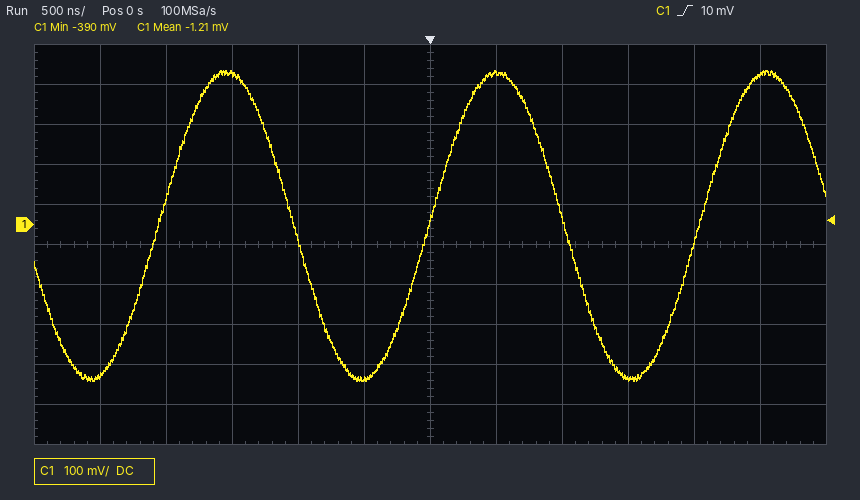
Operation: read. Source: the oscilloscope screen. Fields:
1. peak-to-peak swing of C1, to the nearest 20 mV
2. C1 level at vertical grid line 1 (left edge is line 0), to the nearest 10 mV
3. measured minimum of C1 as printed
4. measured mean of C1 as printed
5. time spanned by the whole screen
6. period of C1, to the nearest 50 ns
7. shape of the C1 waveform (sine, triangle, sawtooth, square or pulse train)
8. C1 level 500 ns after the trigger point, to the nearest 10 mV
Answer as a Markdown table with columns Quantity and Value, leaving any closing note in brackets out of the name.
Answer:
| Quantity | Value |
|---|---|
| peak-to-peak swing of C1, to the nearest 20 mV | 780 mV |
| C1 level at vertical grid line 1 (left edge is line 0), to the nearest 10 mV | -380 mV |
| measured minimum of C1 as printed | -390 mV |
| measured mean of C1 as printed | -1.21 mV |
| time spanned by the whole screen | 6 µs |
| period of C1, to the nearest 50 ns | 2.05 µs |
| shape of the C1 waveform | sine |
| C1 level 500 ns after the trigger point, to the nearest 10 mV | 380 mV |
